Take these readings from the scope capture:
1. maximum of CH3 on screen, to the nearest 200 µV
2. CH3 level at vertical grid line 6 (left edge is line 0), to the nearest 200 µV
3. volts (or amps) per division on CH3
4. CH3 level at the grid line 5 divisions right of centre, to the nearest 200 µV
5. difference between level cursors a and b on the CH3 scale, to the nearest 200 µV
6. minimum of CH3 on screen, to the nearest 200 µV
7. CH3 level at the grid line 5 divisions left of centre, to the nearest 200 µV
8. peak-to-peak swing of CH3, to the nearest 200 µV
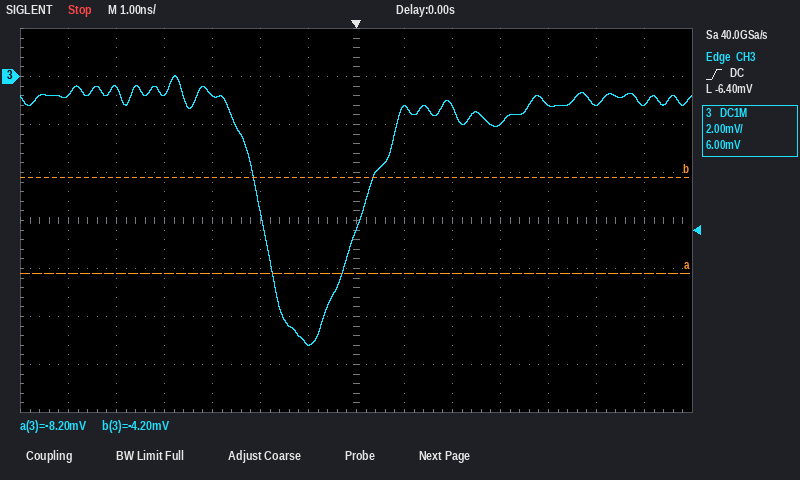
0.0 mV
-11.2 mV
2 mV
-1.2 mV
4.0 mV
-11.2 mV
-400 µV
11.2 mV
